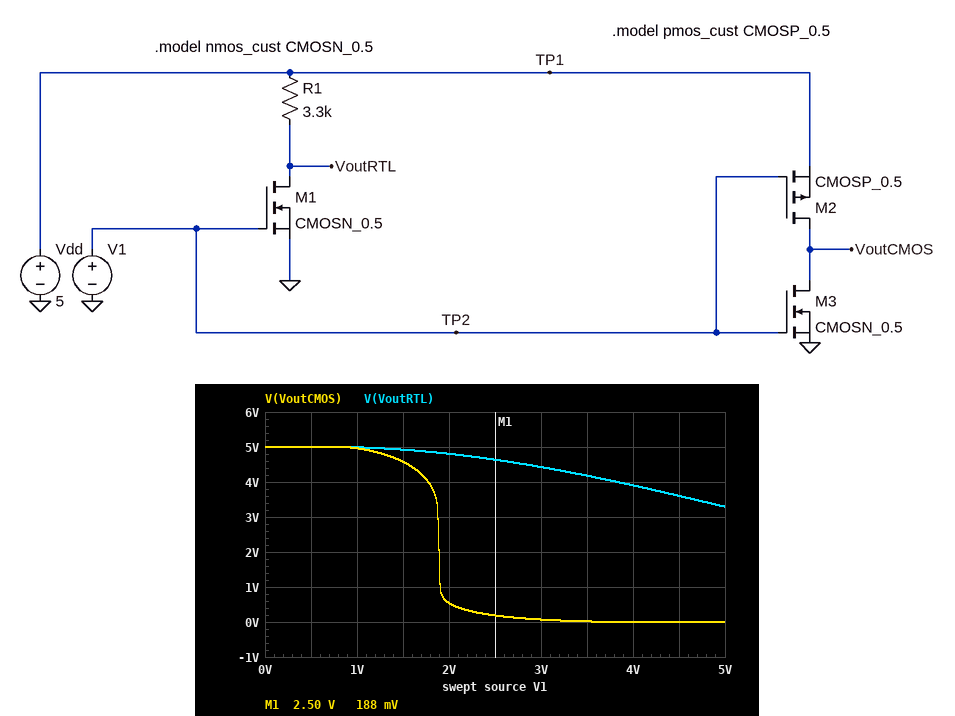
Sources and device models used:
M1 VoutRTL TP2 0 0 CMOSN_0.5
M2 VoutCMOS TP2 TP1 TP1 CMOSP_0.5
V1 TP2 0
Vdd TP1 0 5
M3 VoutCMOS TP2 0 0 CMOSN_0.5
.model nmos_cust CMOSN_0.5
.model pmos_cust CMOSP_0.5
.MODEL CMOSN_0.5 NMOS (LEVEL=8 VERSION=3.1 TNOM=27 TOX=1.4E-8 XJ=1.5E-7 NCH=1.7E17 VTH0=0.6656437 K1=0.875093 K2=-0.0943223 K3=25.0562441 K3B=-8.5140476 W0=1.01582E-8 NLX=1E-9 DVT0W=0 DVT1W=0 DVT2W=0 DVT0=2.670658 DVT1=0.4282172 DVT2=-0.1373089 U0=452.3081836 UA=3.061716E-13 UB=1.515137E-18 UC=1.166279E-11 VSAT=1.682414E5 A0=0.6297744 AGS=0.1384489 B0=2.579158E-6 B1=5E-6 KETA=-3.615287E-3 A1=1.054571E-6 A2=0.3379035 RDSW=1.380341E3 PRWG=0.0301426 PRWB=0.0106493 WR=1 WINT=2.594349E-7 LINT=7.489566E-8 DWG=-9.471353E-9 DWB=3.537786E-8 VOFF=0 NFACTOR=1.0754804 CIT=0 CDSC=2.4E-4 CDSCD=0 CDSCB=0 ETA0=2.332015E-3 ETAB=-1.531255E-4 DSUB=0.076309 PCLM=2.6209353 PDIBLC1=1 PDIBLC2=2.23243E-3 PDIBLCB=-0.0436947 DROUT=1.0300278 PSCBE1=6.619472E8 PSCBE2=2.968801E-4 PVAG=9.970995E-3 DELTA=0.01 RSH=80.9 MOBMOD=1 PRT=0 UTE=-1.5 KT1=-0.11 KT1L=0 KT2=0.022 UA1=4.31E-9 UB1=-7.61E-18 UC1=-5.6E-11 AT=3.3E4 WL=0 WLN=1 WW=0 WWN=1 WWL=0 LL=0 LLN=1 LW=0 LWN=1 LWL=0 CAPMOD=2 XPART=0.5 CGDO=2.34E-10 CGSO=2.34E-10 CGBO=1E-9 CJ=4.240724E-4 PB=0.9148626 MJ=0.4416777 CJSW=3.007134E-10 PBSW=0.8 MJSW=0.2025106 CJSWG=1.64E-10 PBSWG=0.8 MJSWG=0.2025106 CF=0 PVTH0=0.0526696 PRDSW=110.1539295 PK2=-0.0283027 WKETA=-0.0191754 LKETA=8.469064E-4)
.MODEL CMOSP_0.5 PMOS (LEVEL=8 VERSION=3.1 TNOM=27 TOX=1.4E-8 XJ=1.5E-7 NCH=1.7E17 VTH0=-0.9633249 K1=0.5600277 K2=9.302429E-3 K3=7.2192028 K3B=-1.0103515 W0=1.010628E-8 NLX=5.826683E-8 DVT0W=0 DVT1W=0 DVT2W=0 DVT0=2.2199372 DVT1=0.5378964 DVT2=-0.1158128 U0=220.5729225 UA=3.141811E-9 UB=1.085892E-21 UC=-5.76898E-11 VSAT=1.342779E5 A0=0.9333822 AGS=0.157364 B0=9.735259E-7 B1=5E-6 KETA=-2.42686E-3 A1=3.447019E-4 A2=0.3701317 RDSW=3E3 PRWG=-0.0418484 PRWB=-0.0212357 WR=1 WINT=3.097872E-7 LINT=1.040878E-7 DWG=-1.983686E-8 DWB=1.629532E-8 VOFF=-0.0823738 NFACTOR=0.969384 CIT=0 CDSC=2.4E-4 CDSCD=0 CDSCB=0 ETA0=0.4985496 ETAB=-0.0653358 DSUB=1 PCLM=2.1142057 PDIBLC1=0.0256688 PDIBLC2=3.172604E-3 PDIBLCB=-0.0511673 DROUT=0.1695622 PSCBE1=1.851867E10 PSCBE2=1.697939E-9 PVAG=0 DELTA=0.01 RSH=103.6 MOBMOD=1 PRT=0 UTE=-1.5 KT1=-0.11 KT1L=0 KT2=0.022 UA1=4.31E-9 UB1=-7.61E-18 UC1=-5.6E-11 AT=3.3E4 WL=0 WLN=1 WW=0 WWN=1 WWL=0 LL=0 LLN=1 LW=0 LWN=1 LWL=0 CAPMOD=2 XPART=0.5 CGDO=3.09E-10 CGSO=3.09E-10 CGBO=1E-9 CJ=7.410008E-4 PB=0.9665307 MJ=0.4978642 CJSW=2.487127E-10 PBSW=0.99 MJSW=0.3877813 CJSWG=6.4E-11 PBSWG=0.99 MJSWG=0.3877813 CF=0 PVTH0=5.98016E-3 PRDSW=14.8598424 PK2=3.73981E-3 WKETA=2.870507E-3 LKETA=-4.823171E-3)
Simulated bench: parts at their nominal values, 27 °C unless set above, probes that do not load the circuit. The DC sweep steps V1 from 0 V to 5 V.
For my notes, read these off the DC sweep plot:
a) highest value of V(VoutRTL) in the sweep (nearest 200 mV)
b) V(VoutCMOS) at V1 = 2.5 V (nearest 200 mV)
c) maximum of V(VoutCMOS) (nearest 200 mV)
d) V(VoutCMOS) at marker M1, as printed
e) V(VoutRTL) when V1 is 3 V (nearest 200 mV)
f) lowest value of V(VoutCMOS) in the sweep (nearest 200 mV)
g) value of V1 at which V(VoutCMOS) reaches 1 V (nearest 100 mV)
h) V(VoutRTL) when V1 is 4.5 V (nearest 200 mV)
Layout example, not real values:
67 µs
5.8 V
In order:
5.0 V
200 mV
5.0 V
188 mV
4.4 V
0 V
1.9 V
3.6 V
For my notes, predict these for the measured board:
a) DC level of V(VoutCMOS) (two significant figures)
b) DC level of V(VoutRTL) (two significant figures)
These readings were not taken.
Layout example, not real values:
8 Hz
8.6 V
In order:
5.0 V
5.0 V
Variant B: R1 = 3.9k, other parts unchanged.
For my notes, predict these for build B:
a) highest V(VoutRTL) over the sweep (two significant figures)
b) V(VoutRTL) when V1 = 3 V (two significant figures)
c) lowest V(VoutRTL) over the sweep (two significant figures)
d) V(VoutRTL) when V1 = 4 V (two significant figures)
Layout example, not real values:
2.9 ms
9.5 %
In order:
5.0 V
4.3 V
3.0 V
3.7 V
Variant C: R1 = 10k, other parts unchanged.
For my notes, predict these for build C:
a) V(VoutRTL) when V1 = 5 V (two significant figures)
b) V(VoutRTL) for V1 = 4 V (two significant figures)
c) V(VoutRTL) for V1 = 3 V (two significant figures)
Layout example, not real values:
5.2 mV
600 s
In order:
1.5 V
1.9 V
3.3 V
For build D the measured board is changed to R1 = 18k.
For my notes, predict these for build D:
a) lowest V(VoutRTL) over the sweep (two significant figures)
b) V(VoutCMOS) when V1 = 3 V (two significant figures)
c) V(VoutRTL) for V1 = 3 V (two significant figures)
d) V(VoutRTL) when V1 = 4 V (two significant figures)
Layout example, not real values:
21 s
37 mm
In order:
870 mV
70 mV
1.9 V
1.1 V
